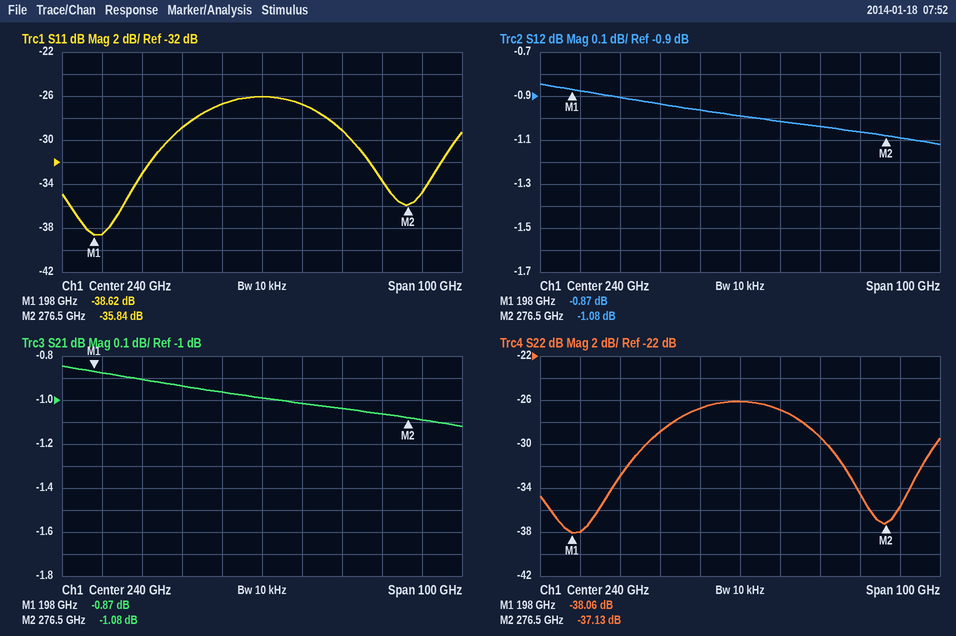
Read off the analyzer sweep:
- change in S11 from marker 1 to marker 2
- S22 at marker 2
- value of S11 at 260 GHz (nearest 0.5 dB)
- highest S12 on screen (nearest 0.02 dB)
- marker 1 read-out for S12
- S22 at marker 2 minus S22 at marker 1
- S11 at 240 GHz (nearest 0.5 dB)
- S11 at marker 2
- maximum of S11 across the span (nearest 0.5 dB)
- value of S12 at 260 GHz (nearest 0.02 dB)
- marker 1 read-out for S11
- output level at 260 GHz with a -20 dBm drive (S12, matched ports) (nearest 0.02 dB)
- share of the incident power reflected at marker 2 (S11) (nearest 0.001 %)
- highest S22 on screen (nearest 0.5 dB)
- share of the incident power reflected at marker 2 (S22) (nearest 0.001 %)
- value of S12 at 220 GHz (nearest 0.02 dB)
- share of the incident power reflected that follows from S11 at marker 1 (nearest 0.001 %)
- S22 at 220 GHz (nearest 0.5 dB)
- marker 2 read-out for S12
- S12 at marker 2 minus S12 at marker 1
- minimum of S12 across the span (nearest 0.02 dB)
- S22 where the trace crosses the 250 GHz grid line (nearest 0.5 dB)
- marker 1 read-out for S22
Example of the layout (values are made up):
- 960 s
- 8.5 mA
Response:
- 2.78 dB
- -37.13 dB
- -29.0 dB
- -0.84 dB
- -0.87 dB
- 0.93 dB
- -26.0 dB
- -35.84 dB
- -26.0 dB
- -1.04 dB
- -38.62 dB
- -21.04 dBm
- 0.026 %
- -26.0 dB
- 0.019 %
- -0.94 dB
- 0.014 %
- -29.0 dB
- -1.08 dB
- -0.21 dB
- -1.12 dB
- -27.0 dB
- -38.06 dB
